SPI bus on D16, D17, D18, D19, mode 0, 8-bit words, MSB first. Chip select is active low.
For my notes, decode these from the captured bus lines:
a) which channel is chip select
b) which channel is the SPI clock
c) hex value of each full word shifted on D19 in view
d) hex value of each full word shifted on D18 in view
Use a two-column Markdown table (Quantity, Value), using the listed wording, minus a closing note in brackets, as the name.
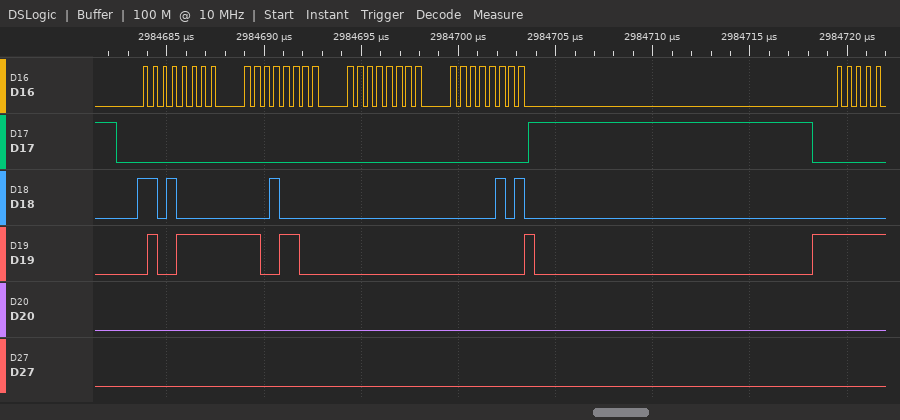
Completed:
| Quantity | Value |
|---|---|
| which channel is chip select | D17 |
| which channel is the SPI clock | D16 |
| hex value of each full word shifted on D19 in view | 4F, CC, 00, 00 |
| hex value of each full word shifted on D18 in view | D0, 10, 00, 05 |
